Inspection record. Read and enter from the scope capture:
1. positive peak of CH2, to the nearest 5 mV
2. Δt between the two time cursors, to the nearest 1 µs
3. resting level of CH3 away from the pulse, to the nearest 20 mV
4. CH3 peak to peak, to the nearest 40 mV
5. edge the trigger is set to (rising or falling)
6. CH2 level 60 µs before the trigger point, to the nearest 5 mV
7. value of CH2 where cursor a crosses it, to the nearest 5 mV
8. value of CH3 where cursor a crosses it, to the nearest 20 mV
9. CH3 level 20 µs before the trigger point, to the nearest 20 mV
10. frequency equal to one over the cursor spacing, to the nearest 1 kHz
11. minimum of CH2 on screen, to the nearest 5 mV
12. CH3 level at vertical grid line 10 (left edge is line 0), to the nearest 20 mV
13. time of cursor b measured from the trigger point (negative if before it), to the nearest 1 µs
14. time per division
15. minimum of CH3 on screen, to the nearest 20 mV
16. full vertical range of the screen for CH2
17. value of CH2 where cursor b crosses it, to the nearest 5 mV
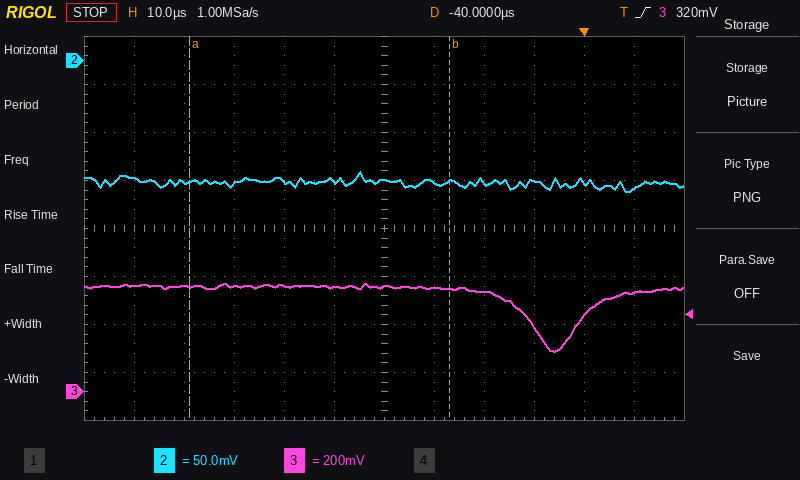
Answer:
-115 mV
52 µs
440 mV
280 mV
rising
-125 mV
-125 mV
440 mV
420 mV
19 kHz
-135 mV
320 mV
-27 µs
10 µs
160 mV
400 mV
-125 mV
